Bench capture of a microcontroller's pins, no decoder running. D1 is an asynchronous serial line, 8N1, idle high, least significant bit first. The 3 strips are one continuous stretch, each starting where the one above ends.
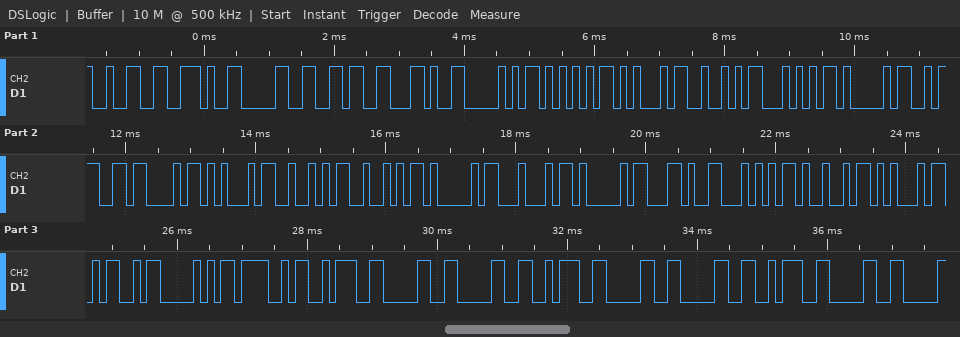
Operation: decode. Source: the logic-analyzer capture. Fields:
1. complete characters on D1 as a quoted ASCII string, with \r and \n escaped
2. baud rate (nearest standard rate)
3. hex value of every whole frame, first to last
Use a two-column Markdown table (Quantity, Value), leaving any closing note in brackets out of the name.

| Quantity | Value |
|---|---|
| complete characters on D1 as a quoted ASCII string, with \r and \n escaped | "2.06,PUERTA:CERRADA,TIEMPO:00:00:0" |
| baud rate | 9600 baud |
| hex value of every whole frame, first to last | 32 2E 30 36 2C 50 55 45 52 54 41 3A 43 45 52 52 41 44 41 2C 54 49 45 4D 50 4F 3A 30 30 3A 30 30 3A 30 |
